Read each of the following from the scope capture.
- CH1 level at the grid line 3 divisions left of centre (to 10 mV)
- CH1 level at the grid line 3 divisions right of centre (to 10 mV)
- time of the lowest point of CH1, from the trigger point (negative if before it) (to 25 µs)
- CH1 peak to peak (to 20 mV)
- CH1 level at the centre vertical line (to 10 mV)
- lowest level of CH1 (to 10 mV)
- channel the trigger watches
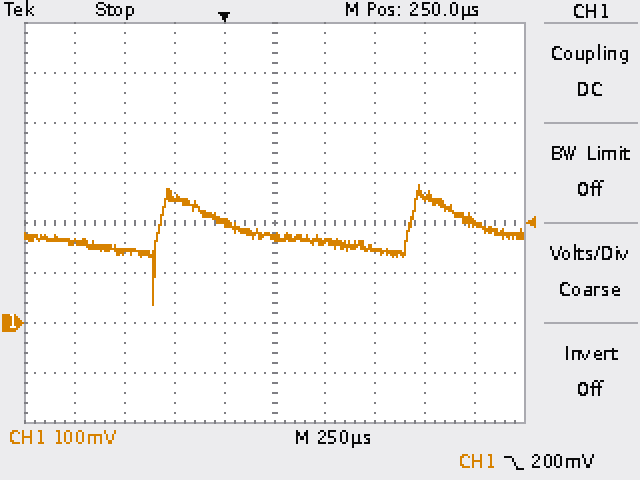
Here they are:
140 mV
250 mV
-350 µs
240 mV
170 mV
40 mV
CH1
